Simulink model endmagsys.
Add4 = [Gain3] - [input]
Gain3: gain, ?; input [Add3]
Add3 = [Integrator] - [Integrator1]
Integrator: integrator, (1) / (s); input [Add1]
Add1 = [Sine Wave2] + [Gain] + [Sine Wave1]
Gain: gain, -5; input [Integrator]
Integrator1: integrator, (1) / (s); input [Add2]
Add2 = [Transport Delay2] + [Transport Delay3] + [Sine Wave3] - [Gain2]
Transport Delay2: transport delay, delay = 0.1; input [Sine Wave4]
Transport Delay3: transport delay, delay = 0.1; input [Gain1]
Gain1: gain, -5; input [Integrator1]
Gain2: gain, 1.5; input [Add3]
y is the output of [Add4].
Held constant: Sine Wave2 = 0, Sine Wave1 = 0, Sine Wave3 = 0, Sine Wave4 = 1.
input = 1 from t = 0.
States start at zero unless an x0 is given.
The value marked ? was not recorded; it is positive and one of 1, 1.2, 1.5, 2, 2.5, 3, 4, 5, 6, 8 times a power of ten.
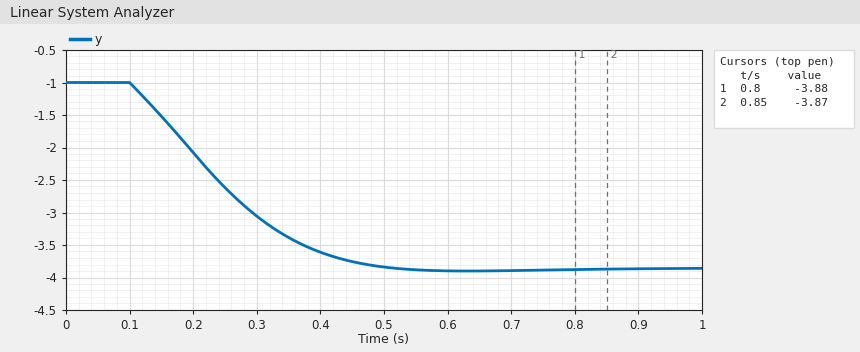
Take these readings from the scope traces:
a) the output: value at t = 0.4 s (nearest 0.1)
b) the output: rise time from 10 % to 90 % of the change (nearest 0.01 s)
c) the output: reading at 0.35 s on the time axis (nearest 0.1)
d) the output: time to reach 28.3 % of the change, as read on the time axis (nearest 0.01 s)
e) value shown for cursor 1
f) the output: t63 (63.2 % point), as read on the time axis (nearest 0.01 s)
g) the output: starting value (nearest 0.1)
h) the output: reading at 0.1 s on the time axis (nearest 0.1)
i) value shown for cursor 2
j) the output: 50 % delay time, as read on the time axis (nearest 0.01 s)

-3.6
0.26 s
-3.4
0.18 s
-3.88
0.27 s
-1.0
-1.0
-3.87
0.23 s
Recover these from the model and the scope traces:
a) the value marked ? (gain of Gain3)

10
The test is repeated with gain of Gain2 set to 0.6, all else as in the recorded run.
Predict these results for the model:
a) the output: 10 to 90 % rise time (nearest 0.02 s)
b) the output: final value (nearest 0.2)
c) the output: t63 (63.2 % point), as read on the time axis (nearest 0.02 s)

0.22 s
-3.2
0.24 s
